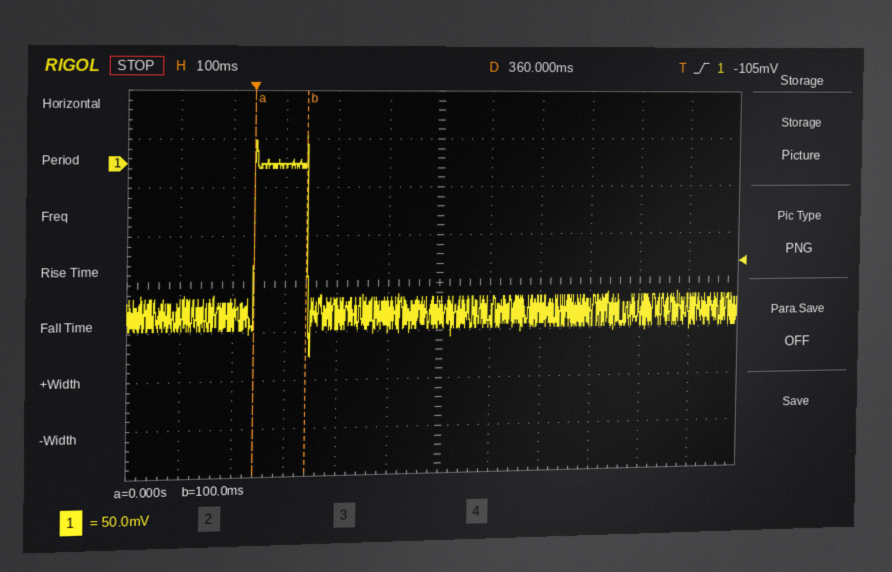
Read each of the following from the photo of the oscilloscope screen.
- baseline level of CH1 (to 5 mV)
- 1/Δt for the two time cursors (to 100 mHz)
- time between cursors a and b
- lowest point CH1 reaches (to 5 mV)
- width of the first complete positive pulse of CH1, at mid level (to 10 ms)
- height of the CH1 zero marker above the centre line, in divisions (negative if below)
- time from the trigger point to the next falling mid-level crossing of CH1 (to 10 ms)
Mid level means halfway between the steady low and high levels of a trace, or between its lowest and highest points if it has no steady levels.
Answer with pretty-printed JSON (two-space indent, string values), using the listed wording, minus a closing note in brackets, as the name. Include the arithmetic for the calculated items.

{
  "baseline level of CH1": "-155 mV",
  "1/Δt for the two time cursors": "1 / 100 ms ≈ 10.0 Hz",
  "time between cursors a and b": "100 ms − (0 s) = 100 ms",
  "lowest point CH1 reaches": "-200 mV",
  "width of the first complete positive pulse of CH1, at mid level": "100 ms",
  "height of the CH1 zero marker above the centre line, in divisions": "+2.5 div",
  "time from the trigger point to the next falling mid-level crossing of CH1": "100 ms"
}
